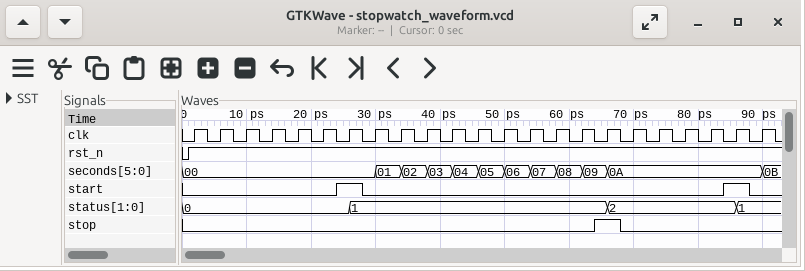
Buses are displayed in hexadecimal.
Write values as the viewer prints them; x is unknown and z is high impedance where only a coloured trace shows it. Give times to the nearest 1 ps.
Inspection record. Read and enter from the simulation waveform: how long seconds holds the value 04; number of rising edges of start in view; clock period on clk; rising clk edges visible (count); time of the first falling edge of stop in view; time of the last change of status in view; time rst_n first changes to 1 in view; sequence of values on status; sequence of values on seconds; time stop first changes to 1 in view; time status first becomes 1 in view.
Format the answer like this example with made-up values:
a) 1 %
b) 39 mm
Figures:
a) 4 ps
b) 2
c) 4 ps
d) 23
e) 68 ps
f) 86 ps
g) 1 ps
h) 0, 1, 2, 1
i) 00, 01, 02, 03, 04, 05, 06, 07, 08, 09, 0A, 0B
j) 64 ps
k) 26 ps
